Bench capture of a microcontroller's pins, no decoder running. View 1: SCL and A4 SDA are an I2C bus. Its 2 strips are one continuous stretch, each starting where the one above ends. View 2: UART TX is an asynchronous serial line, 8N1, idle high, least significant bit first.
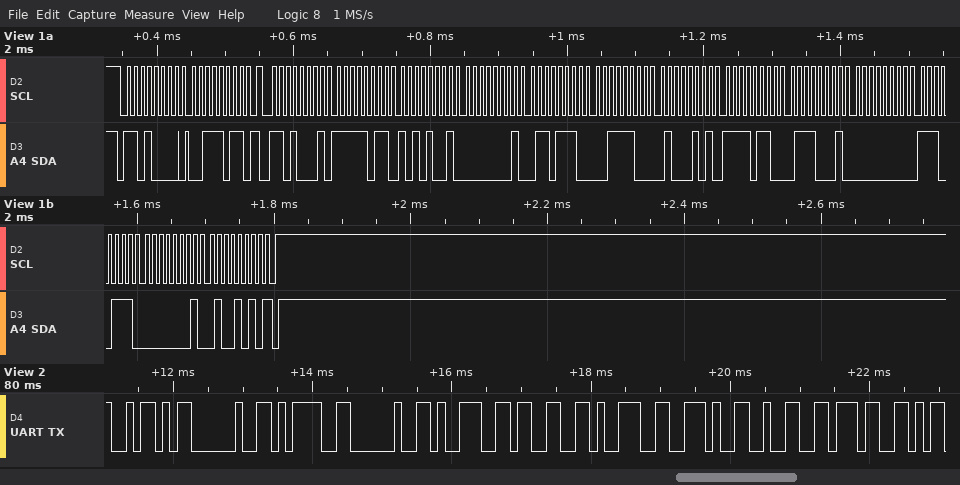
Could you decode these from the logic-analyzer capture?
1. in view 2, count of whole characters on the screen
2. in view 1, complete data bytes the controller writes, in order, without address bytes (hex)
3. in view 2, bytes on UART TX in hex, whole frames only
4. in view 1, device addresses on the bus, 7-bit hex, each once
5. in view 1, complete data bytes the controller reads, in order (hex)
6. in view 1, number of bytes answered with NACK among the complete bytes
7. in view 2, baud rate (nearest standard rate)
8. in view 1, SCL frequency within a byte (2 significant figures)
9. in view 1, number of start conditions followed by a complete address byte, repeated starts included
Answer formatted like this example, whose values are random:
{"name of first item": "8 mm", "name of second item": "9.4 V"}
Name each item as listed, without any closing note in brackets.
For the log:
{"in view 2, count of whole characters on the screen": "10", "in view 1, complete data bytes the controller writes, in order, without address bytes": "3B", "in view 2, bytes on UART TX in hex, whole frames only": "5A 20 3D 20 39 33 39 2E 32 37", "in view 1, device addresses on the bus, 7-bit hex, each once": "0x68", "in view 1, complete data bytes the controller reads, in order": "FB A9 01 6E 3C 45 F6 71 00 E7 01 4A", "in view 1, number of bytes answered with NACK among the complete bytes": "1", "in view 2, baud rate": "9600 baud", "in view 1, SCL frequency within a byte": "100 kHz", "in view 1, number of start conditions followed by a complete address byte, repeated starts included": "2"}
